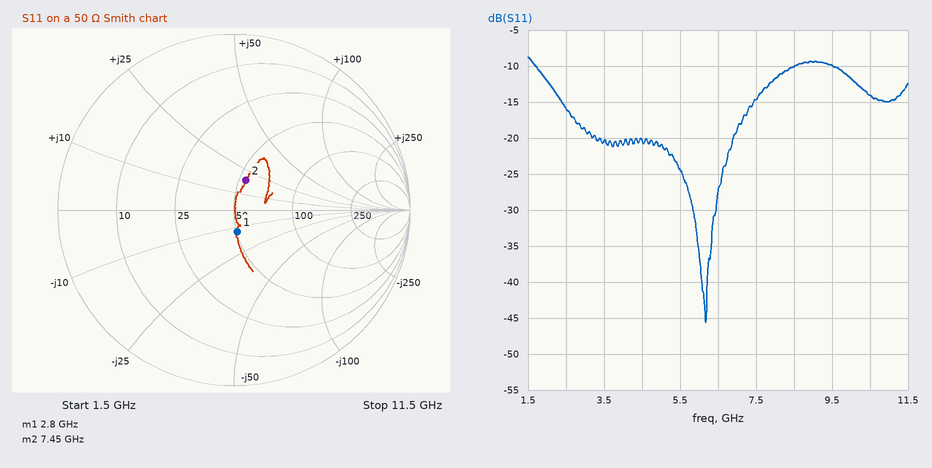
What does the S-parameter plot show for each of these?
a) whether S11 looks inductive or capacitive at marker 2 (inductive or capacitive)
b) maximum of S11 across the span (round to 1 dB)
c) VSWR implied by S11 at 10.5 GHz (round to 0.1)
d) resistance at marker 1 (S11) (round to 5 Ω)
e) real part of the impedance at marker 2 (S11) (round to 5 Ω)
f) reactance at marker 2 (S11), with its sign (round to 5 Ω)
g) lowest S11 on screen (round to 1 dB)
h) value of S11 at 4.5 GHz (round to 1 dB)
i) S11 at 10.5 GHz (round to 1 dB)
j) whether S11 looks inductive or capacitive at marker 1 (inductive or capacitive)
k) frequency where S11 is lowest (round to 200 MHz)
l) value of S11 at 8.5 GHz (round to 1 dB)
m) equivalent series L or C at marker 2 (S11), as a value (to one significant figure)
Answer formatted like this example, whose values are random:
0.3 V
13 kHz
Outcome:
inductive
-9 dB
1.5
50 Ω
55 Ω
+20 Ω
-46 dB
-20 dB
-14 dB
capacitive
6.2 GHz
-10 dB
400 pH
